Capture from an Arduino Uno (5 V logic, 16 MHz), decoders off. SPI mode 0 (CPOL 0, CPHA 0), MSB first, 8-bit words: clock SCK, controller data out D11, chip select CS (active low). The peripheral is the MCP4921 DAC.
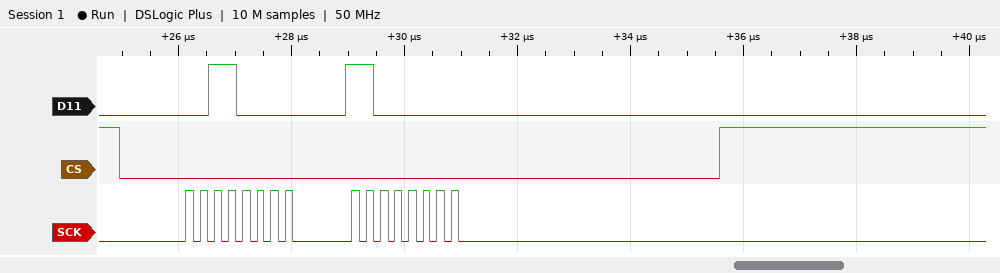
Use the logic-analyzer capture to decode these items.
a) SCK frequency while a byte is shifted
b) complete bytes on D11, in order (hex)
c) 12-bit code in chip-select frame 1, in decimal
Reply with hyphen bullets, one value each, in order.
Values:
- 4 MHz
- 30 C0
- 192
